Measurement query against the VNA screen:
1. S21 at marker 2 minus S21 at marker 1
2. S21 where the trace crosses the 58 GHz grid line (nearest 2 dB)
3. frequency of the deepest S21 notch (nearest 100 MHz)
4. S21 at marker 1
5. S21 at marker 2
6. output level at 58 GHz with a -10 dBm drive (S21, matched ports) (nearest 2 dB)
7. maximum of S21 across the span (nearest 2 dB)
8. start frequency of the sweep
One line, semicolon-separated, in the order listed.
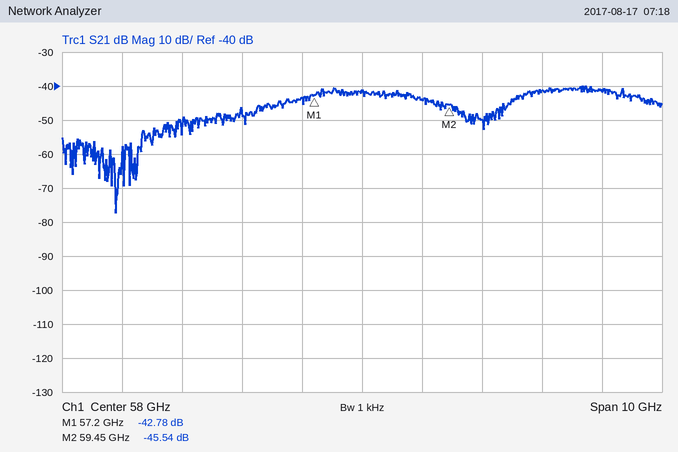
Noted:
-2.76 dB; -42 dB; 53.9 GHz; -42.78 dB; -45.54 dB; -52 dBm; -40 dB; 53 GHz
